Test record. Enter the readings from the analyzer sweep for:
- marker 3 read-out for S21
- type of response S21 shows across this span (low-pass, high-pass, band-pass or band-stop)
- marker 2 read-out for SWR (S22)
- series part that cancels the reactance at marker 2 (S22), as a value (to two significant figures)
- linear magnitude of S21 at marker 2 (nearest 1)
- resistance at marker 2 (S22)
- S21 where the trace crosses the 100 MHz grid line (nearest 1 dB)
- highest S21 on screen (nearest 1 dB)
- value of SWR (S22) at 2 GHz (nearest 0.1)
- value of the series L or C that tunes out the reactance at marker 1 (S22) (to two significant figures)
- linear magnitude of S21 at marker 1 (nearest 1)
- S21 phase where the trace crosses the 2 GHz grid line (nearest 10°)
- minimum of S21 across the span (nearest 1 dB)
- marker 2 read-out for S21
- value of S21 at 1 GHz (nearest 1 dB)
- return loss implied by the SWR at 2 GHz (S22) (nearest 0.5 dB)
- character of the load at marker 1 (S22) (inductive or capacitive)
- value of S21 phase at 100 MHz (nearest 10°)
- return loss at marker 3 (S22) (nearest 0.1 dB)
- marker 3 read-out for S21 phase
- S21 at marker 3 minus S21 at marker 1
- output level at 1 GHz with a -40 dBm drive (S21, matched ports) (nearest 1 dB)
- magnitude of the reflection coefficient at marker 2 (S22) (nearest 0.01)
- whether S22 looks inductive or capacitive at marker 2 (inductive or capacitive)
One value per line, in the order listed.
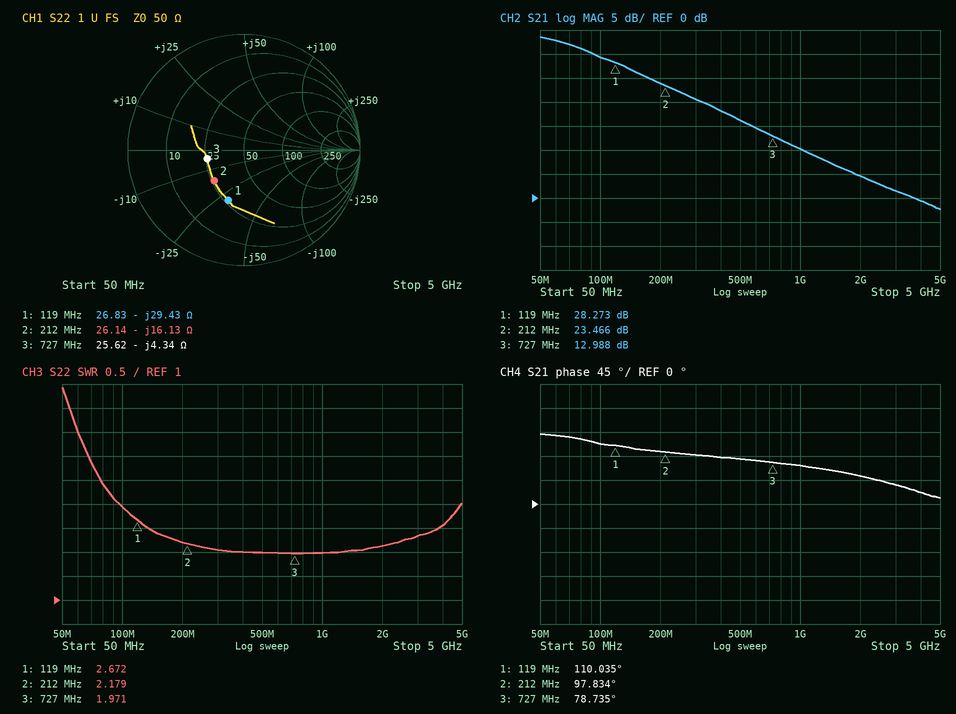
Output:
12.988 dB
low-pass
2.179
12 nH
15
26.14 Ω
29 dB
34 dB
2.1
39 nH
26
50°
-2 dB
23.466 dB
10 dB
9.0 dB
capacitive
110°
9.7 dB
78.735°
-15.285 dB
-30 dBm
0.37
capacitive
